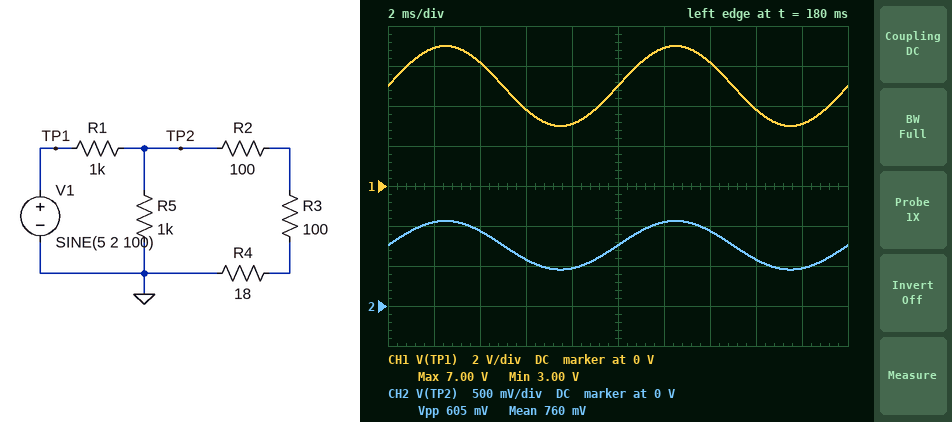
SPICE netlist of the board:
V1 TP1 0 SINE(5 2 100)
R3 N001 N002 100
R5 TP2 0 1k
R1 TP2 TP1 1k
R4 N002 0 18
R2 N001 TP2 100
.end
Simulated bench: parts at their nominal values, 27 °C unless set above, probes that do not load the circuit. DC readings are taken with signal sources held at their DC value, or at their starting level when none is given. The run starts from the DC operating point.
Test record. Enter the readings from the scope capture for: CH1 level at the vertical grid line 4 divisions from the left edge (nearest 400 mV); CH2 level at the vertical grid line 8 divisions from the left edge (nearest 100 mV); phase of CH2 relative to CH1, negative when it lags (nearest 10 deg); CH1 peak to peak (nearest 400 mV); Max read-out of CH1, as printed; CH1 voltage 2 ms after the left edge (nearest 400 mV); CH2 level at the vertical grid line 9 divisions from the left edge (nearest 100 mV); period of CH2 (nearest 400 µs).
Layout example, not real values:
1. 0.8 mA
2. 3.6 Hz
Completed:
1. 3.2 V
2. 600 mV
3. 0 deg
4. 4.0 V
5. 7.00 V
6. 6.8 V
7. 500 mV
8. 10.0 ms
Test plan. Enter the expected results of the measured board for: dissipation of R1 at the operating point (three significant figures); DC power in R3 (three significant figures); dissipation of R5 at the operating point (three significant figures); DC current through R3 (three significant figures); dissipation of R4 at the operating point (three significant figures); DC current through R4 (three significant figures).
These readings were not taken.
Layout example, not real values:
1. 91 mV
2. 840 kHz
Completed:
1. 18.0 mW
2. 1.21 mW
3. 576 µW
4. 3.48 mA
5. 218 µW
6. 3.48 mA
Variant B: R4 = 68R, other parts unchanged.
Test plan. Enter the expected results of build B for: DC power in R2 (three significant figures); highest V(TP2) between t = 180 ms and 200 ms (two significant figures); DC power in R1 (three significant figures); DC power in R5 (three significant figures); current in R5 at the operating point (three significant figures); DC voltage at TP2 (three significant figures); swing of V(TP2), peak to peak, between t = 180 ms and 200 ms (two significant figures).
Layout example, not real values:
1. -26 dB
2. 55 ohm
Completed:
1. 1.06 mW
2. 1.2 V
3. 17.0 mW
4. 761 µW
5. 872 µA
6. 872 mV
7. 700 mV
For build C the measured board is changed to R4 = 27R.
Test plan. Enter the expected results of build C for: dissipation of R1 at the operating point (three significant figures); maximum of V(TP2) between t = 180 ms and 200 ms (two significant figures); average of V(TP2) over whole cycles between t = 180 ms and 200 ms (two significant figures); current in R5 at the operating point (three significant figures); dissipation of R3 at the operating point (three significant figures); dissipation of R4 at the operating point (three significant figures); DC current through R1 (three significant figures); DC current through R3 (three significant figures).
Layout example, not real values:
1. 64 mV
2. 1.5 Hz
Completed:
1. 17.8 mW
2. 1.1 V
3. 780 mV
4. 781 µA
5. 1.18 mW
6. 319 µW
7. 4.22 mA
8. 3.44 mA
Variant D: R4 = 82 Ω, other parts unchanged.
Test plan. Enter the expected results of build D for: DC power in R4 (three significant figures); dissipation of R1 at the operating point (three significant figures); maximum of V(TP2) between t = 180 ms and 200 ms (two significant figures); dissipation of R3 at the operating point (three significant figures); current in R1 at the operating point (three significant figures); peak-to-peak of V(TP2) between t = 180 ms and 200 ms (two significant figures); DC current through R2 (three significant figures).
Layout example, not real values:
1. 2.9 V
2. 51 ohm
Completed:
1. 838 µW
2. 16.8 mW
3. 1.3 V
4. 1.02 mW
5. 4.10 mA
6. 720 mV
7. 3.20 mA
